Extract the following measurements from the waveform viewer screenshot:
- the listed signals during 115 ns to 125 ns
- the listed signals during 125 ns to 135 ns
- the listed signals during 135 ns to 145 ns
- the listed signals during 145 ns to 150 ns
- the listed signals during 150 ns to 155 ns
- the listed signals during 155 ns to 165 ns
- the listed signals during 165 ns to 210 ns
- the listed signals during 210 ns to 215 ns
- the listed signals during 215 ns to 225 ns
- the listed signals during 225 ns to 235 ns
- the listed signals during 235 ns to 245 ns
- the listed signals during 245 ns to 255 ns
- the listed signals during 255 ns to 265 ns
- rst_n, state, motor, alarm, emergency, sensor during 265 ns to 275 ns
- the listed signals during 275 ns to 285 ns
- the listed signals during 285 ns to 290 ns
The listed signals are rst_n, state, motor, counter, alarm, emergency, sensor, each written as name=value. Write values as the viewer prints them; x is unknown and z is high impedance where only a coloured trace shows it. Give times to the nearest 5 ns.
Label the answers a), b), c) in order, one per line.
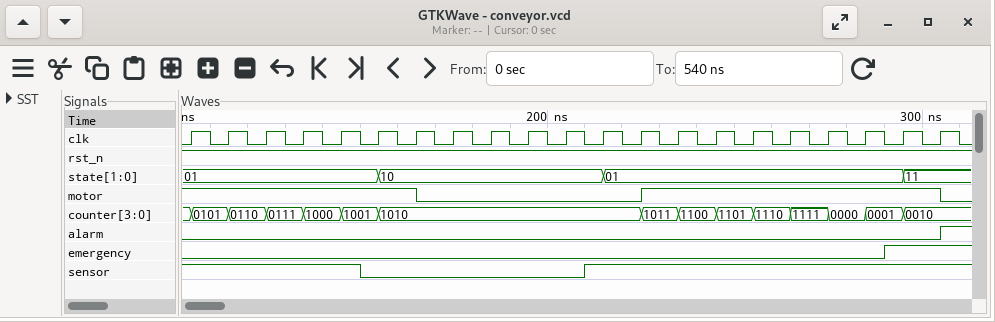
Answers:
a) rst_n=1, state=01, motor=1, counter=0110, alarm=0, emergency=0, sensor=1
b) rst_n=1, state=01, motor=1, counter=0111, alarm=0, emergency=0, sensor=1
c) rst_n=1, state=01, motor=1, counter=1000, alarm=0, emergency=0, sensor=1
d) rst_n=1, state=01, motor=1, counter=1001, alarm=0, emergency=0, sensor=1
e) rst_n=1, state=01, motor=1, counter=1001, alarm=0, emergency=0, sensor=0
f) rst_n=1, state=10, motor=1, counter=1010, alarm=0, emergency=0, sensor=0
g) rst_n=1, state=10, motor=0, counter=1010, alarm=0, emergency=0, sensor=0
h) rst_n=1, state=10, motor=0, counter=1010, alarm=0, emergency=0, sensor=1
i) rst_n=1, state=01, motor=0, counter=1010, alarm=0, emergency=0, sensor=1
j) rst_n=1, state=01, motor=1, counter=1011, alarm=0, emergency=0, sensor=1
k) rst_n=1, state=01, motor=1, counter=1100, alarm=0, emergency=0, sensor=1
l) rst_n=1, state=01, motor=1, counter=1101, alarm=0, emergency=0, sensor=1
m) rst_n=1, state=01, motor=1, counter=1110, alarm=0, emergency=0, sensor=1
n) rst_n=1, state=01, motor=1, alarm=0, emergency=0, sensor=1
o) rst_n=1, state=01, motor=1, counter=0000, alarm=0, emergency=0, sensor=1
p) rst_n=1, state=01, motor=1, counter=0001, alarm=0, emergency=0, sensor=1
